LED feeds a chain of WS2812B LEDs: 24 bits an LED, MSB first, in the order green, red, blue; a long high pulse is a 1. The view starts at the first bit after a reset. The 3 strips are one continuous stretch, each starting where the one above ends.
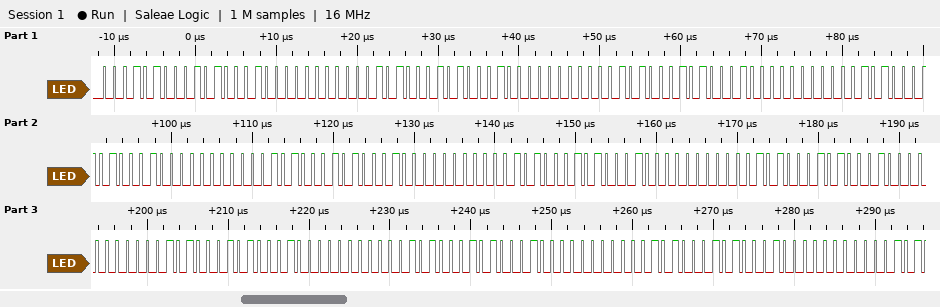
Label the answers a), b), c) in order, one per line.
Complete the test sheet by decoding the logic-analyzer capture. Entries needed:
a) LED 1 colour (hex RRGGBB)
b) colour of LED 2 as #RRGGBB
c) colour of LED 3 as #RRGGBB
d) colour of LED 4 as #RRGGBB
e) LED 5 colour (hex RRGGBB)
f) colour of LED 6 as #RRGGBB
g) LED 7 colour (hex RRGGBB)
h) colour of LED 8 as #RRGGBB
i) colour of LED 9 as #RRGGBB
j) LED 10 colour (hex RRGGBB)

a) #511400
b) #511400
c) #511400
d) #511400
e) #511400
f) #511400
g) #511400
h) #511400
i) #511400
j) #511400
